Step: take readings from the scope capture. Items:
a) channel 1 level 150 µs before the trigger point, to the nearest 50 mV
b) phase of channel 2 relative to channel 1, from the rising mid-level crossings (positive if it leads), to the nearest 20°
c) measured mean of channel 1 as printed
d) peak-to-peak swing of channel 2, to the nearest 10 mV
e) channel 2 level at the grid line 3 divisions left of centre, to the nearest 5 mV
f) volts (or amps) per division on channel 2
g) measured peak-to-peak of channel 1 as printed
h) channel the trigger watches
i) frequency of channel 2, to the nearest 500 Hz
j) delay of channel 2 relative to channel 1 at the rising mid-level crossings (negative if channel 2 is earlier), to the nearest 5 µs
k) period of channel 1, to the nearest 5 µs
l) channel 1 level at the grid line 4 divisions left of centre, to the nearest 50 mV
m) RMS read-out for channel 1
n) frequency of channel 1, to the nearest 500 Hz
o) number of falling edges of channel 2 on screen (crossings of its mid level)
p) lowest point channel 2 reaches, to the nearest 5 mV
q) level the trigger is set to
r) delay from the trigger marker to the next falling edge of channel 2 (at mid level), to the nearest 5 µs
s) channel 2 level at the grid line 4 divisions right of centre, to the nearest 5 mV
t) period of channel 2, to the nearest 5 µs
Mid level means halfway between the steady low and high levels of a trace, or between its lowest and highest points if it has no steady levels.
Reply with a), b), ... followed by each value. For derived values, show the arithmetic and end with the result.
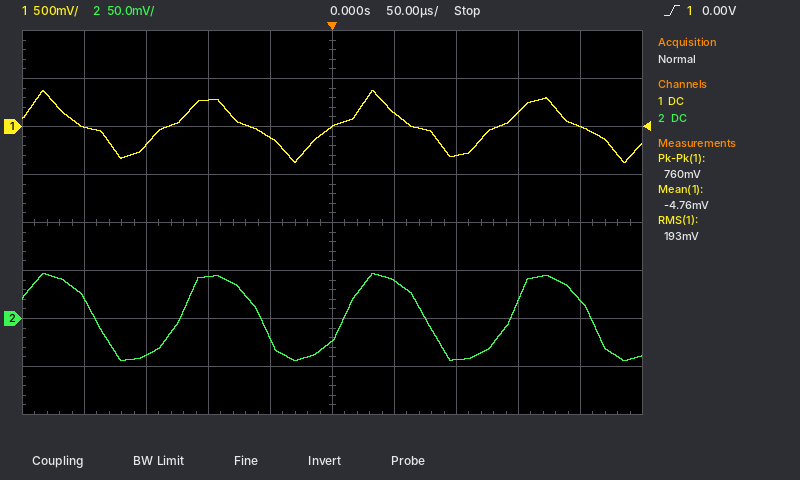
a) -200 mV
b) −360° × (+10 µs) / 135 µs ≈ -26.7°, so -20° to the nearest 20°
c) -4.76 mV
d) 90 mV
e) -40 mV
f) 50 mV
g) 760 mV
h) channel 1
i) 1 / 135 µs ≈ 7.41 kHz, so 7.5 kHz to the nearest 500 Hz
j) +10 µs
k) 135 µs
l) 0 mV
m) 193 mV
n) 1 / 135 µs ≈ 7.41 kHz, so 7.5 kHz to the nearest 500 Hz
o) 4
p) -45 mV
q) 0.00 V
r) 75 µs
s) 20 mV
t) 135 µs
